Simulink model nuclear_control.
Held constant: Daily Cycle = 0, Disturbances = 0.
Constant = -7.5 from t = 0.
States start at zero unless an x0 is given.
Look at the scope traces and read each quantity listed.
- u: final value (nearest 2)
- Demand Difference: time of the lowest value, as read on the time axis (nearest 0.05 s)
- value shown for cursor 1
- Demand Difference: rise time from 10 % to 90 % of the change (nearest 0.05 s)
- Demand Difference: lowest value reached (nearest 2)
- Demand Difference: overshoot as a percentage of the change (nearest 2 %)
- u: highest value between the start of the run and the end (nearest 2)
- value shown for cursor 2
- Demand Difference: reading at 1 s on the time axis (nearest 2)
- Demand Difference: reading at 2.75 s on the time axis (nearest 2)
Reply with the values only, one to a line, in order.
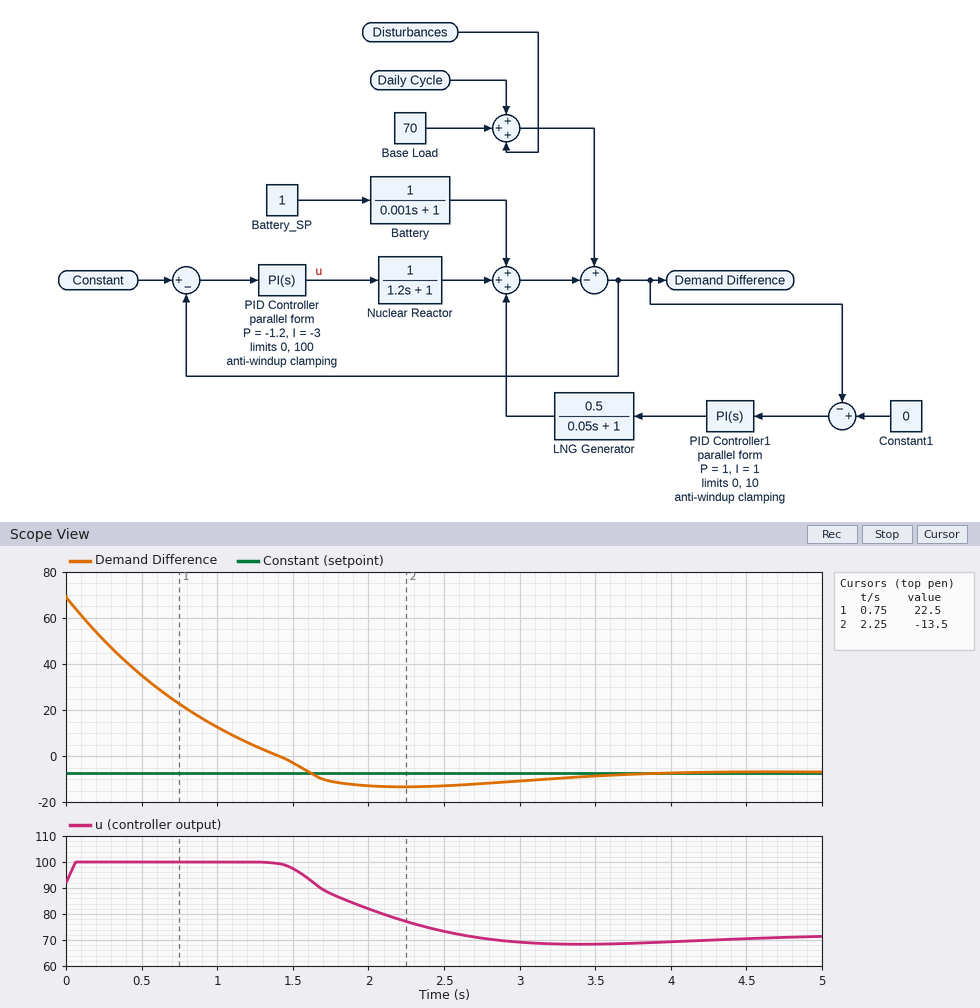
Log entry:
72
2.25 s
22.5
1.30 s
-14
8 %
100
-13.5
12
-12
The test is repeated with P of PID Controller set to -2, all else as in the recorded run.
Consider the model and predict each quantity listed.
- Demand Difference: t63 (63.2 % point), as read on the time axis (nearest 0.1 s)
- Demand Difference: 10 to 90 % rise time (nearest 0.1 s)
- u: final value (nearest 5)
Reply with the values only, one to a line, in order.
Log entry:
0.8 s
1.4 s
70
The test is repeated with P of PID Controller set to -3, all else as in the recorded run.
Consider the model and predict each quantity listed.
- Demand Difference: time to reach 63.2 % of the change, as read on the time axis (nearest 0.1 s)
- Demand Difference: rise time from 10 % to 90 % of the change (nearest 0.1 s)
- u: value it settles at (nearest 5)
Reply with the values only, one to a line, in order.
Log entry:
0.8 s
1.7 s
70
